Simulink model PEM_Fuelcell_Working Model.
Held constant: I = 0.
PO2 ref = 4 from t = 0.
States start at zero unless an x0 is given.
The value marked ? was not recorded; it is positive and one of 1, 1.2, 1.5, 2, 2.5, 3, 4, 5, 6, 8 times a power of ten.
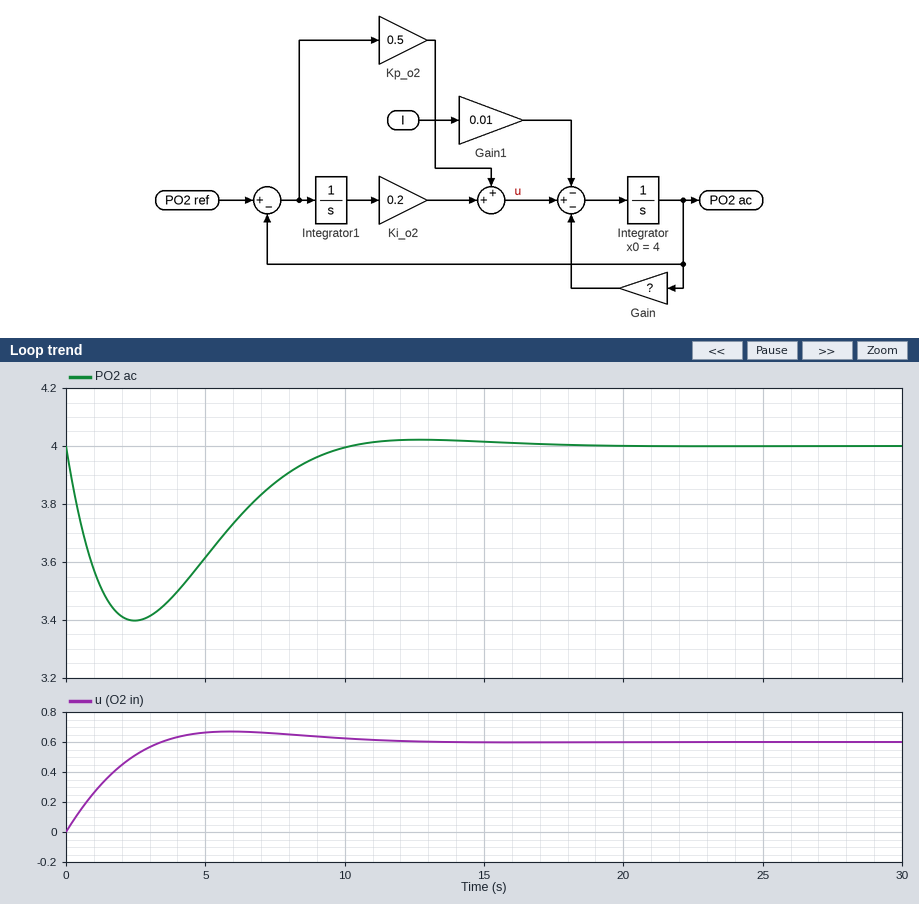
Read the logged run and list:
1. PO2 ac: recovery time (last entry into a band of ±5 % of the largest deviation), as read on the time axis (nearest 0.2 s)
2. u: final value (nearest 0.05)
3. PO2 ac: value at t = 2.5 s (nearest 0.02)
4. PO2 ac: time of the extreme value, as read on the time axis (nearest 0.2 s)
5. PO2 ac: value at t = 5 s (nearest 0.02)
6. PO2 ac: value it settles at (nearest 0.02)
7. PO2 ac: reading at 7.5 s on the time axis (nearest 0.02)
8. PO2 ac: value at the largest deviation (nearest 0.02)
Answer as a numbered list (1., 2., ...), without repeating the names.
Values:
1. 9.2 s
2. 0.60
3. 3.40
4. 2.4 s
5. 3.62
6. 4.00
7. 3.88
8. 3.40
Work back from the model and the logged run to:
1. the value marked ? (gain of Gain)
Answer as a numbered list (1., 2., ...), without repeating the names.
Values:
1. 0.15
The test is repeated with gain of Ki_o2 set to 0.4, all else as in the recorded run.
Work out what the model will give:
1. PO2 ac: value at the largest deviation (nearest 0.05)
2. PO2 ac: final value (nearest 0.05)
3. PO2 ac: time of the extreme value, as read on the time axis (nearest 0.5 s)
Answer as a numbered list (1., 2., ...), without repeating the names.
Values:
1. 3.50
2. 4.00
3. 2.0 s
